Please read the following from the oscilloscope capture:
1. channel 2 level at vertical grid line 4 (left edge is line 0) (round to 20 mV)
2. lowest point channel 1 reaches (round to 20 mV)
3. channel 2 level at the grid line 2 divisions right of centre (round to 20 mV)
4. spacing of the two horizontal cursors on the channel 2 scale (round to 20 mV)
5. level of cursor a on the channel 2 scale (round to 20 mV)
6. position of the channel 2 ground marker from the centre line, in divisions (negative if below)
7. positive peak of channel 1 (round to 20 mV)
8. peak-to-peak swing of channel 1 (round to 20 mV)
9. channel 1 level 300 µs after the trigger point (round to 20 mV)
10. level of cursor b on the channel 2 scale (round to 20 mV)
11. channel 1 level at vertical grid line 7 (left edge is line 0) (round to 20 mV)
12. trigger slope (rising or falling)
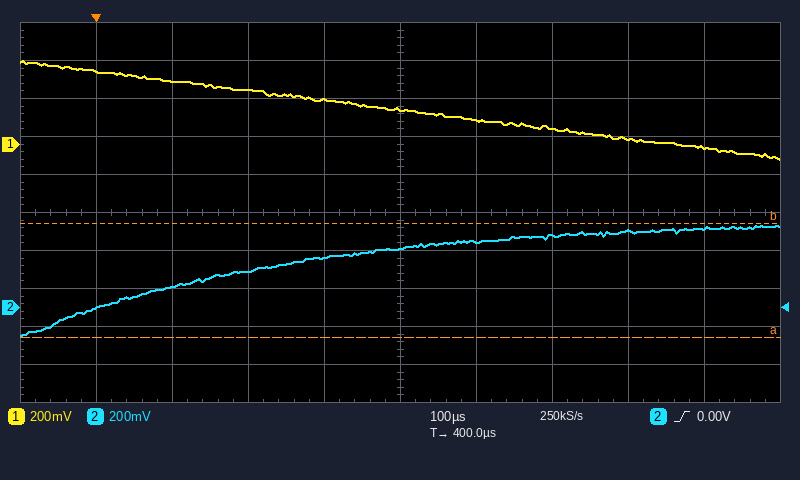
260 mV
-80 mV
380 mV
600 mV
-160 mV
-2.5 div
440 mV
520 mV
240 mV
440 mV
80 mV
rising
